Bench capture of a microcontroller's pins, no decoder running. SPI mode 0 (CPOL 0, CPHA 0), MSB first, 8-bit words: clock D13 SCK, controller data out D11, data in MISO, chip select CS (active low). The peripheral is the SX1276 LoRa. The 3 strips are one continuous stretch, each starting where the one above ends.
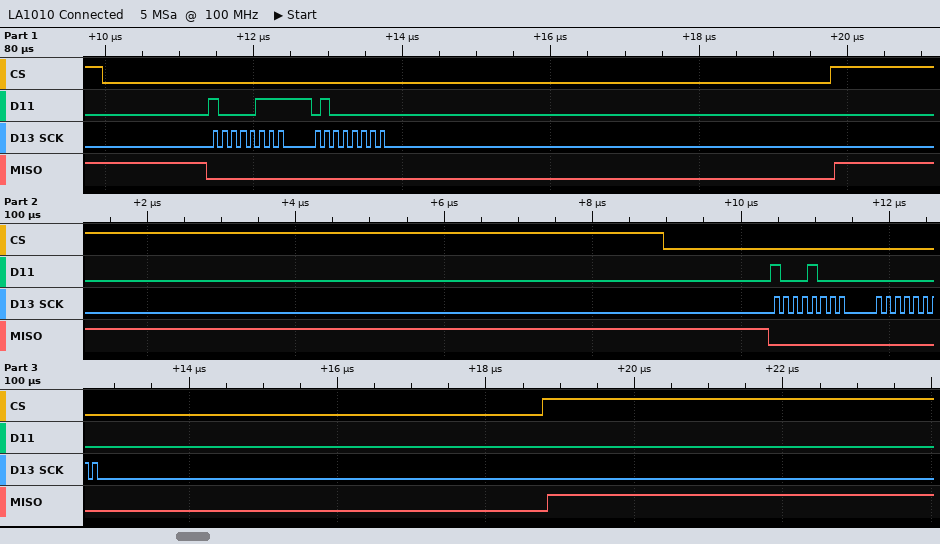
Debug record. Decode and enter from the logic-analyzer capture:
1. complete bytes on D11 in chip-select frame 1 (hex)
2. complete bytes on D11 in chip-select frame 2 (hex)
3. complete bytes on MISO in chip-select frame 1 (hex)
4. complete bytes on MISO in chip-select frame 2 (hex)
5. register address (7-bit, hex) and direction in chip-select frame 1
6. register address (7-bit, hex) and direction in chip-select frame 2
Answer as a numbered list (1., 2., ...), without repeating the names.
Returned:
1. 87 40
2. 88 00
3. 00 00
4. 00 00
5. 0x07 write
6. 0x08 write
